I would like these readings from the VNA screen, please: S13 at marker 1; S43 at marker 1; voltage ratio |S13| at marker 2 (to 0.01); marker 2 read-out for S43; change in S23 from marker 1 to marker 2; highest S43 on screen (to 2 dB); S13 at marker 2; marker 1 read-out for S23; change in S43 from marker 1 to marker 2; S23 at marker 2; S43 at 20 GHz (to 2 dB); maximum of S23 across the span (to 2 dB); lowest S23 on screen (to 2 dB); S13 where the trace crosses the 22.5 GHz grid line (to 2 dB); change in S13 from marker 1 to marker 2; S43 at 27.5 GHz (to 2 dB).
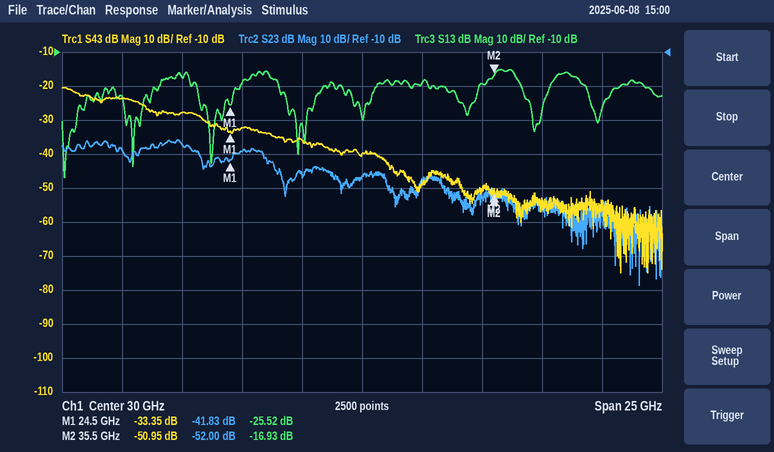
-25.52 dB
-33.35 dB
0.14
-50.95 dB
-10.17 dB
-20 dB
-16.93 dB
-41.83 dB
-17.60 dB
-52.00 dB
-24 dB
-36 dB
-78 dB
-18 dB
8.59 dB
-36 dB
